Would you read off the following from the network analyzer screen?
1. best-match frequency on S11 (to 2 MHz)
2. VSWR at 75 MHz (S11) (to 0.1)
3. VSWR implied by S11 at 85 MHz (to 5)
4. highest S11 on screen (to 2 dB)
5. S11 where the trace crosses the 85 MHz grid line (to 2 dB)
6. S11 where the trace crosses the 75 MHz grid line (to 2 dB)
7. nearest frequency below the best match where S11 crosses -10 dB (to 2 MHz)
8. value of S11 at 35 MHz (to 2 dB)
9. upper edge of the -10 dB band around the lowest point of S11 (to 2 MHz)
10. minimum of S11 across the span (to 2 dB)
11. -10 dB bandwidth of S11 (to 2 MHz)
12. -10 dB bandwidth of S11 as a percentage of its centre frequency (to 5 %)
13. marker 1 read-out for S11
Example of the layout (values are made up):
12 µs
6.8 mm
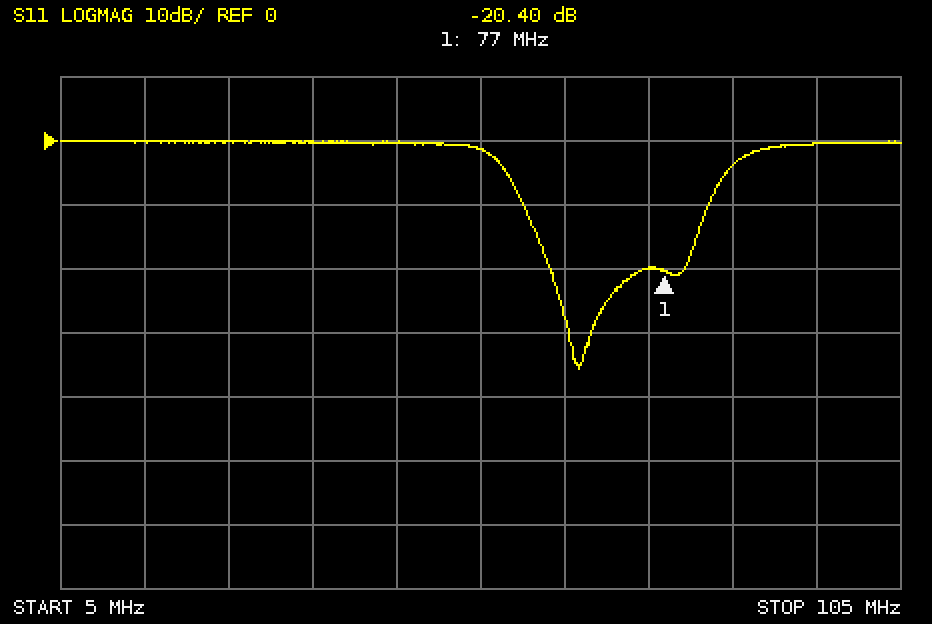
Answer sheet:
66 MHz
1.2
5
0 dB
-4 dB
-20 dB
60 MHz
0 dB
82 MHz
-36 dB
22 MHz
30 %
-20.40 dB
